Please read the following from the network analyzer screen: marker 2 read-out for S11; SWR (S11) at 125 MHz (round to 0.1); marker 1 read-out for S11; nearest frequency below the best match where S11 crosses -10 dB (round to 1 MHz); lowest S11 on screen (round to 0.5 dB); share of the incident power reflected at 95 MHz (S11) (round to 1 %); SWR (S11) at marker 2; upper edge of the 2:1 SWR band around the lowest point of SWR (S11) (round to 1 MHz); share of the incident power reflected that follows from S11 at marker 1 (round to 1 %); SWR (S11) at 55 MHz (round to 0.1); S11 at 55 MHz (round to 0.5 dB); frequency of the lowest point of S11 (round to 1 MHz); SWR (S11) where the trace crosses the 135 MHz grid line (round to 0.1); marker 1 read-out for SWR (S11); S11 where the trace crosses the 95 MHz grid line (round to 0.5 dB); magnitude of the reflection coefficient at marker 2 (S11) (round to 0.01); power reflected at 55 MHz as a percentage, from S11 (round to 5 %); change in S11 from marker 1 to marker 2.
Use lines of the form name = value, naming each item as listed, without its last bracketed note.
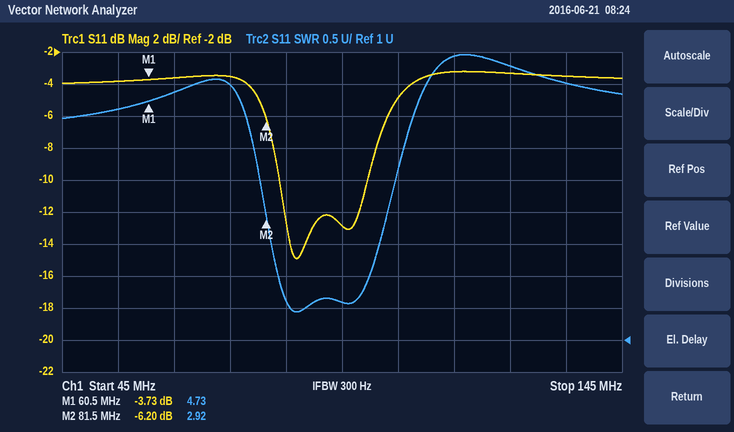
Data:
marker 2 read-out for S11 = -6.20 dB
SWR (S11) at 125 MHz = 5.3
marker 1 read-out for S11 = -3.73 dB
nearest frequency below the best match where S11 crosses -10 dB = 84 MHz
lowest S11 on screen = -15.0 dB
share of the incident power reflected at 95 MHz (S11) = 5 %
SWR (S11) at marker 2 = 2.92
upper edge of the 2:1 SWR band around the lowest point of SWR (S11) = 100 MHz
share of the incident power reflected that follows from S11 at marker 1 = 42 %
SWR (S11) at 55 MHz = 4.6
S11 at 55 MHz = -4.0 dB
frequency of the lowest point of S11 = 87 MHz
SWR (S11) where the trace crosses the 135 MHz grid line = 5.0
marker 1 read-out for SWR = 4.73
S11 where the trace crosses the 95 MHz grid line = -13.0 dB
magnitude of the reflection coefficient at marker 2 (S11) = 0.49
power reflected at 55 MHz as a percentage, from S11 = 40 %
change in S11 from marker 1 to marker 2 = -2.47 dB
